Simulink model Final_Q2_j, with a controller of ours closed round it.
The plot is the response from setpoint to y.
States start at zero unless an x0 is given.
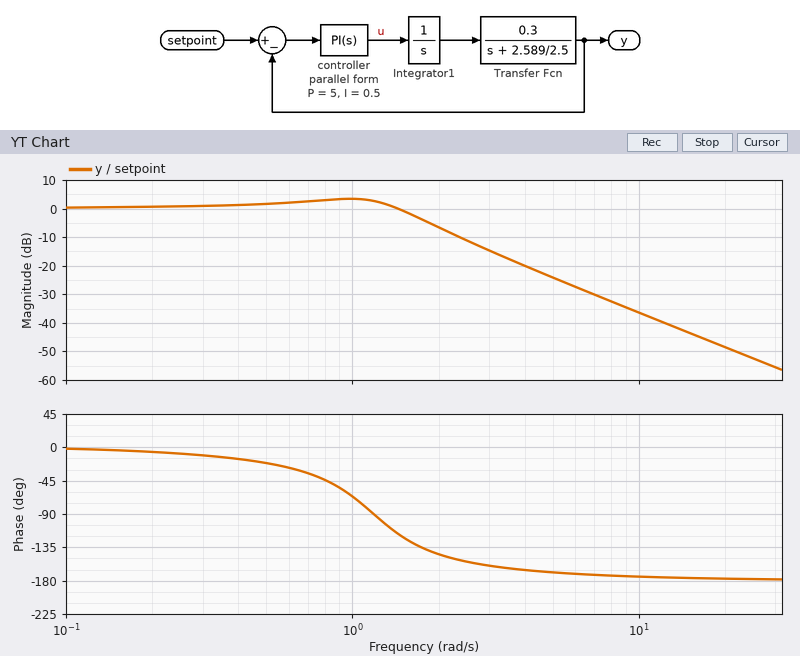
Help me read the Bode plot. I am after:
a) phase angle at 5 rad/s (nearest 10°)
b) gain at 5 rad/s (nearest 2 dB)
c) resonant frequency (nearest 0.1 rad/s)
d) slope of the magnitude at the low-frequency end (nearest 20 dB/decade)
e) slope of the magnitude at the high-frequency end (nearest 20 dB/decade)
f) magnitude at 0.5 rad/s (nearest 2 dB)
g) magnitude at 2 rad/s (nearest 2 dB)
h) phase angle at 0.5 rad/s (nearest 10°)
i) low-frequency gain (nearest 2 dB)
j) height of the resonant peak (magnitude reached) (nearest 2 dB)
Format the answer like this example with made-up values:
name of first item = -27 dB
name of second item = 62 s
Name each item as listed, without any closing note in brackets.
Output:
phase angle at 5 rad/s = -170°
gain at 5 rad/s = -24 dB
resonant frequency = 1.0 rad/s
slope of the magnitude at the low-frequency end = 0 dB/decade
slope of the magnitude at the high-frequency end = -40 dB/decade
magnitude at 0.5 rad/s = 2 dB
magnitude at 2 rad/s = -6 dB
phase angle at 0.5 rad/s = -20°
low-frequency gain = 0 dB
height of the resonant peak (magnitude reached) = 4 dB
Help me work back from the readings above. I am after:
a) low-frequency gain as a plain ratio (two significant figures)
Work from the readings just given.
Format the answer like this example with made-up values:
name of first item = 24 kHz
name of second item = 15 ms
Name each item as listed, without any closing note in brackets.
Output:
low-frequency gain as a plain ratio = 1.0
